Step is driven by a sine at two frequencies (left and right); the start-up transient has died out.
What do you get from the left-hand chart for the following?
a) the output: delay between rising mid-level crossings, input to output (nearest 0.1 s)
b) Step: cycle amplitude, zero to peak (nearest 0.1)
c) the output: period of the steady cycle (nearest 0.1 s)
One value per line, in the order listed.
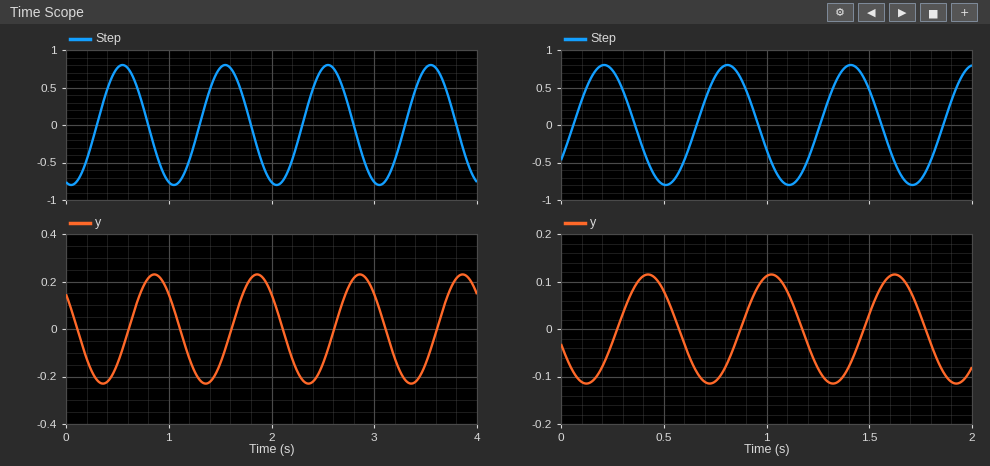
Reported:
0.3 s
0.8
1.0 s
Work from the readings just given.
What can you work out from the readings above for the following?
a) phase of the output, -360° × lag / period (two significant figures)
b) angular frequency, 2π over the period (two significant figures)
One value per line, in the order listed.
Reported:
-110°
6.3 rad/s
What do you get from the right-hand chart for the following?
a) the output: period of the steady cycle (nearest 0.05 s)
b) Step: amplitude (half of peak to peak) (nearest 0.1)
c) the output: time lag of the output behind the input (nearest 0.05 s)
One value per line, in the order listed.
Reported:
0.60 s
0.8
0.20 s
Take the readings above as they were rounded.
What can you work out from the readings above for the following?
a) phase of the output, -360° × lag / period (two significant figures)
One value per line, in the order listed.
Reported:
-120°
